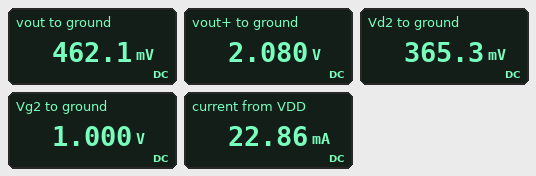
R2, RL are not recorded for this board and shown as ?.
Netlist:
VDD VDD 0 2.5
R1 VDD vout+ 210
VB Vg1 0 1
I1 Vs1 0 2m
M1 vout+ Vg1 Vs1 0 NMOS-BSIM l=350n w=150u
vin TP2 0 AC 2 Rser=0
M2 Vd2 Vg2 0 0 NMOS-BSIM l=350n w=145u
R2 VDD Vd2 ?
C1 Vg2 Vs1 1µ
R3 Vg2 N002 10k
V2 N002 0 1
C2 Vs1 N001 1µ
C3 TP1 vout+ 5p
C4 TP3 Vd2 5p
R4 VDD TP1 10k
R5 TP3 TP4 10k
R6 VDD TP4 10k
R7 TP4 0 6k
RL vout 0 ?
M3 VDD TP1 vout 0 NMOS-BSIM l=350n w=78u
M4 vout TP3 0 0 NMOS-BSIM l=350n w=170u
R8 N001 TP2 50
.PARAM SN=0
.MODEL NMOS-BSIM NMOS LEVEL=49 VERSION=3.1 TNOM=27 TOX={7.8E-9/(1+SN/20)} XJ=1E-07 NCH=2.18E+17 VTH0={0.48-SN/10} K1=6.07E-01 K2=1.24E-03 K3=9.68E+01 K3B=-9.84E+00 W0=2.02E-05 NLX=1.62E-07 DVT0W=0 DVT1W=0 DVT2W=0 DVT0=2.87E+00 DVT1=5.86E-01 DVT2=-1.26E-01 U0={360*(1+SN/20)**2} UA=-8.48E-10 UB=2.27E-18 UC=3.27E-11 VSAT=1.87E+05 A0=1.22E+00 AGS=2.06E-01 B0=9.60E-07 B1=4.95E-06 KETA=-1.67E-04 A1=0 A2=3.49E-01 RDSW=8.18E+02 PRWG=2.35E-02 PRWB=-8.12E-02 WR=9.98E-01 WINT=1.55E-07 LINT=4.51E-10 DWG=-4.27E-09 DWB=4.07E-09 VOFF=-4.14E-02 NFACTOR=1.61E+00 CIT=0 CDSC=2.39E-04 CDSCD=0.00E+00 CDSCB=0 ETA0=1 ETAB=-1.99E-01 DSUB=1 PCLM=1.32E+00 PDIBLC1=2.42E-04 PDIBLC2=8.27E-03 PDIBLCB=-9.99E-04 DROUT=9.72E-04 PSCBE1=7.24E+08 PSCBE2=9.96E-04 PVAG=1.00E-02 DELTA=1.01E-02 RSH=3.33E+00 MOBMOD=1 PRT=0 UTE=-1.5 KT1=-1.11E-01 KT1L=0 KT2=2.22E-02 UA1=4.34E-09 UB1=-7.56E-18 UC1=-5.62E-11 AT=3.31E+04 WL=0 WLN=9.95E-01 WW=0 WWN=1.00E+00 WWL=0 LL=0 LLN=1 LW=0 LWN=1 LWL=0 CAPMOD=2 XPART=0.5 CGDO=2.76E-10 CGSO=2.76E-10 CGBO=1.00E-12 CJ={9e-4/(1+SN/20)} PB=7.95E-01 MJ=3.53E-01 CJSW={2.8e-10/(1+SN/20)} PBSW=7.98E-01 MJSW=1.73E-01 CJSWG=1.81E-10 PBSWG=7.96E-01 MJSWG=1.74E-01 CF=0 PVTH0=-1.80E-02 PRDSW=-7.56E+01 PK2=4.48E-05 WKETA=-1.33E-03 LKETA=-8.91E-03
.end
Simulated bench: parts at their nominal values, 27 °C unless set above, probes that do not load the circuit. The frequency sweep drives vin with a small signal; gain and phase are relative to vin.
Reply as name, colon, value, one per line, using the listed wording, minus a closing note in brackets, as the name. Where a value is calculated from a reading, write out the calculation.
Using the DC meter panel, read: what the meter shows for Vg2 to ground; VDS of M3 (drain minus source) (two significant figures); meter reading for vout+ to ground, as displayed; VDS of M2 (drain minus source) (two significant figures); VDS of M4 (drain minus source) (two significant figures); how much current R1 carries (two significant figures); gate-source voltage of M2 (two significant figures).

what the meter shows for Vg2 to ground: 1.000 V
VDS of M3 (drain minus source): 2.5 V - 462.1 mV = 2.0 V
meter reading for vout+ to ground, as displayed: 2.080 V
VDS of M2 (drain minus source): 365.3 mV = 370 mV
VDS of M4 (drain minus source): 462.1 mV = 460 mV
how much current R1 carries: (2.5 V - 2.08 V) / 210 Ω = 2.0 mA
gate-source voltage of M2: 1 V = 1.0 V
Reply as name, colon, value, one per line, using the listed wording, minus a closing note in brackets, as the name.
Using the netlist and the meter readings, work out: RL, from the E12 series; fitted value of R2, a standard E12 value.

RL, from the E12 series: 39 Ω
fitted value of R2, a standard E12 value: 470 Ω
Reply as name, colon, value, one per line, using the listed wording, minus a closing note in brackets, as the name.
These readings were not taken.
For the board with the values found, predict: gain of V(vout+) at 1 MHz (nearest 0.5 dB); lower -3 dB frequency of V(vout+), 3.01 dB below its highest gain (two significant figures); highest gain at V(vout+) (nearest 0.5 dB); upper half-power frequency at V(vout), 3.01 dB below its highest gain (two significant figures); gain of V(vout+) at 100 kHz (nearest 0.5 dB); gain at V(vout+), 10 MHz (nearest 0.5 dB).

gain of V(vout+) at 1 MHz: 6.0 dB
lower -3 dB frequency of V(vout+), 3.01 dB below its highest gain: 1.5 kHz
highest gain at V(vout+): 6.0 dB
upper half-power frequency at V(vout), 3.01 dB below its highest gain: 2.9 GHz
gain of V(vout+) at 100 kHz: 6.0 dB
gain at V(vout+), 10 MHz: 6.0 dB
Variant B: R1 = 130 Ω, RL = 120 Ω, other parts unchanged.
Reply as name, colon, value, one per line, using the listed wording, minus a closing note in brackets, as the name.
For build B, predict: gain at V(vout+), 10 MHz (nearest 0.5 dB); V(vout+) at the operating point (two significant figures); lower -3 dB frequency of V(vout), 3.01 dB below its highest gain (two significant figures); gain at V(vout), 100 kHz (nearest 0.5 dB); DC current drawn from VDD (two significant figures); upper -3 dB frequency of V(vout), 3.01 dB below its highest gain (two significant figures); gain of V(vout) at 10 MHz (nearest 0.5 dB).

gain at V(vout+), 10 MHz: 2.0 dB
V(vout+) at the operating point: 2.2 V
lower -3 dB frequency of V(vout), 3.01 dB below its highest gain: 2.5 MHz
gain at V(vout), 100 kHz: -23.0 dB
DC current drawn from VDD: 18 mA
upper -3 dB frequency of V(vout), 3.01 dB below its highest gain: 2.7 GHz
gain of V(vout) at 10 MHz: 4.5 dB
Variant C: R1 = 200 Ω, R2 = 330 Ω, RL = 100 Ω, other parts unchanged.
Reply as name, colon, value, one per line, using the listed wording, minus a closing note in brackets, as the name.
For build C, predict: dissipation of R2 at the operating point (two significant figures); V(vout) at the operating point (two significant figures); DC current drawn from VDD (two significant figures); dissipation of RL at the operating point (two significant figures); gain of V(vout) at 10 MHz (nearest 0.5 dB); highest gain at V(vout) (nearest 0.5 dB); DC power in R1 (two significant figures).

dissipation of R2 at the operating point: 8.7 mW
V(vout) at the operating point: 720 mV
DC current drawn from VDD: 19 mA
dissipation of RL at the operating point: 5.1 mW
gain of V(vout) at 10 MHz: 8.5 dB
highest gain at V(vout): 9.0 dB
DC power in R1: 800 µW
